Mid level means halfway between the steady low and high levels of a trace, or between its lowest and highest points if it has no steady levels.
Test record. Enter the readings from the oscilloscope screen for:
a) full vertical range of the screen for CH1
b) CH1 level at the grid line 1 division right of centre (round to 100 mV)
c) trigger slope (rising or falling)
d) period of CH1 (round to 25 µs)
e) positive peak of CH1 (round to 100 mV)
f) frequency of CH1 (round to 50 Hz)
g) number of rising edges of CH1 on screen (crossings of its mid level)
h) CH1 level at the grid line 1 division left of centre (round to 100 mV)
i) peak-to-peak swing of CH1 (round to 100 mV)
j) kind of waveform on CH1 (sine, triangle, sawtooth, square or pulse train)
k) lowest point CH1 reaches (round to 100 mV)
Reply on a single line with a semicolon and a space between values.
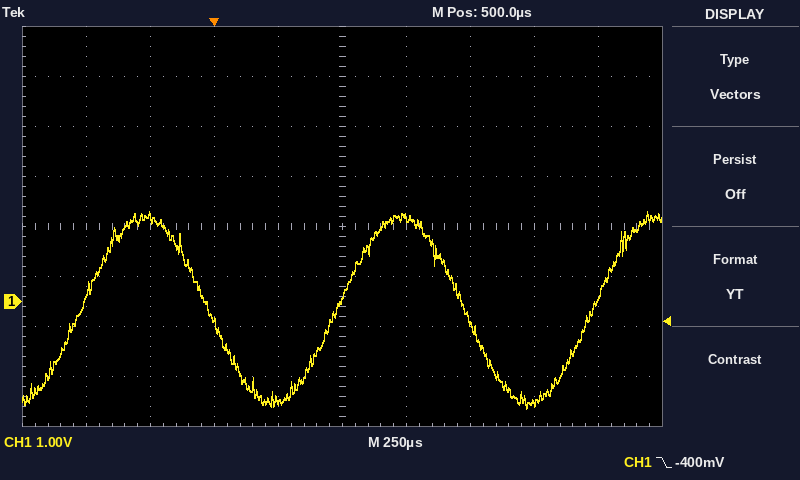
8 V; 1.7 V; falling; 1.000 ms; 1.8 V; 1.00 kHz; 3; -2.0 V; 3.9 V; sine; -2.1 V
